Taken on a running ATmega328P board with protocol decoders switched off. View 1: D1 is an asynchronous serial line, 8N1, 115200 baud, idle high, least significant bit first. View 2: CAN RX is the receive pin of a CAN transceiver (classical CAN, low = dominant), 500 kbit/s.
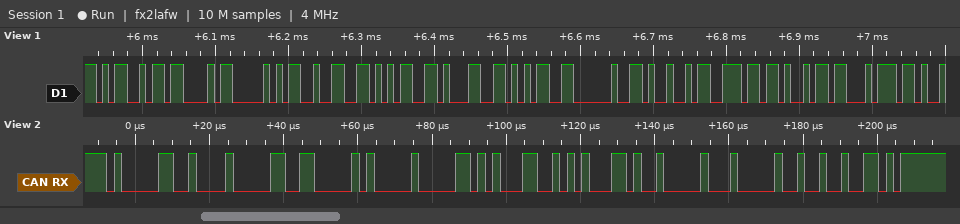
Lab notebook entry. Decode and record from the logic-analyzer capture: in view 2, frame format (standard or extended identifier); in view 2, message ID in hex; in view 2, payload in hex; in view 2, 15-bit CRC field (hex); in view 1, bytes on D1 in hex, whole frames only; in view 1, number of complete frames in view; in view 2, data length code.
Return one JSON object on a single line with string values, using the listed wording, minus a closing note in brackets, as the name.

{"in view 2, frame format": "standard", "in view 2, message ID in hex": "0x412", "in view 2, payload in hex": "26 04 00 A8 CA 8D 20 10", "in view 2, 15-bit CRC field": "0x0926", "in view 1, bytes on D1 in hex, whole frames only": "4D 43 50 32 35 31 35 20 49 6E 69 74", "in view 1, number of complete frames in view": "12", "in view 2, data length code": "8"}
